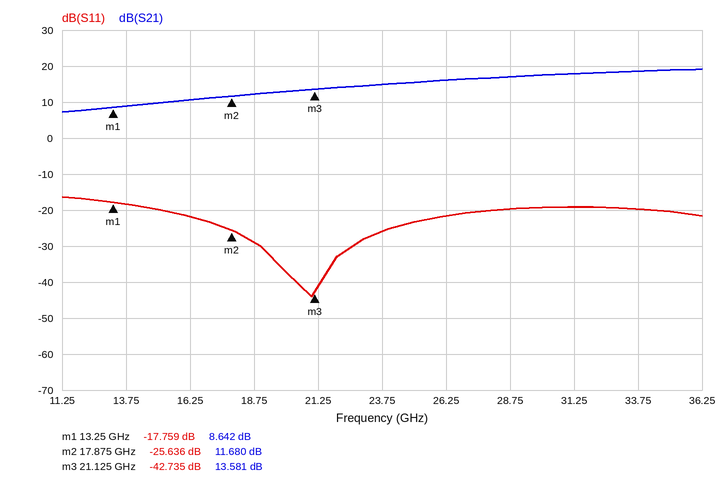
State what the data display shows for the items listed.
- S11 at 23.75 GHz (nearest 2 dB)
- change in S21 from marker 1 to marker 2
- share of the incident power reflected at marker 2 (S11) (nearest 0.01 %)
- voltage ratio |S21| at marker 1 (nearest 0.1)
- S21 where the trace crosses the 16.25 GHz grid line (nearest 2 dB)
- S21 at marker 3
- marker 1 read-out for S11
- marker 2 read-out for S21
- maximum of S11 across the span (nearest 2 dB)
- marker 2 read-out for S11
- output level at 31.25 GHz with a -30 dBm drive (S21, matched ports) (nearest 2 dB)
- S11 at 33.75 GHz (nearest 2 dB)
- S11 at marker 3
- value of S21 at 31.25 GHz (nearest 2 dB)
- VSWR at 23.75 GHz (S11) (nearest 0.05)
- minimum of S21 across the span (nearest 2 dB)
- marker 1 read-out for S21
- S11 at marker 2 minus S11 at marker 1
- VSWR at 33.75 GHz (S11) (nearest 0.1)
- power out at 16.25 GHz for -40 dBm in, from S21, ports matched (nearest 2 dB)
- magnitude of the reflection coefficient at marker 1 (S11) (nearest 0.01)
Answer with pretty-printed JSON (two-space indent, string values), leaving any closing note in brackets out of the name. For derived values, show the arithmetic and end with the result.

{
  "S11 at 23.75 GHz": "-26 dB",
  "change in S21 from marker 1 to marker 2": "11.68 − (8.642) = 3.038 dB",
  "share of the incident power reflected at marker 2 (S11)": "10^(-25.636/10) ≈ 0.27 %",
  "voltage ratio |S21| at marker 1": "10^(8.642/20) ≈ 2.7",
  "S21 where the trace crosses the 16.25 GHz grid line": "10 dB",
  "S21 at marker 3": "13.581 dB",
  "marker 1 read-out for S11": "-17.759 dB",
  "marker 2 read-out for S21": "11.680 dB",
  "maximum of S11 across the span": "-16 dB",
  "marker 2 read-out for S11": "-25.636 dB",
  "output level at 31.25 GHz with a -30 dBm drive (S21, matched ports)": "-30 dBm + (18 dB) = -12 dBm",
  "S11 at 33.75 GHz": "-20 dB",
  "S11 at marker 3": "-42.735 dB",
  "value of S21 at 31.25 GHz": "18 dB",
  "VSWR at 23.75 GHz (S11)": "|Γ| = 10^(-26/20) = 0.0501; VSWR = (1 + 0.0501)/(1 − 0.0501) ≈ 1.11, so 1.10 to the nearest 0.05",
  "minimum of S21 across the span": "8 dB",
  "marker 1 read-out for S21": "8.642 dB",
  "S11 at marker 2 minus S11 at marker 1": "-25.636 − (-17.759) = -7.877 dB",
  "VSWR at 33.75 GHz (S11)": "|Γ| = 10^(-20/20) = 0.1000; VSWR = (1 + 0.1000)/(1 − 0.1000) ≈ 1.2",
  "power out at 16.25 GHz for -40 dBm in, from S21, ports matched": "-40 dBm + (10 dB) = -30 dBm",
  "magnitude of the reflection coefficient at marker 1 (S11)": "10^(-17.759/20) ≈ 0.13"
}
